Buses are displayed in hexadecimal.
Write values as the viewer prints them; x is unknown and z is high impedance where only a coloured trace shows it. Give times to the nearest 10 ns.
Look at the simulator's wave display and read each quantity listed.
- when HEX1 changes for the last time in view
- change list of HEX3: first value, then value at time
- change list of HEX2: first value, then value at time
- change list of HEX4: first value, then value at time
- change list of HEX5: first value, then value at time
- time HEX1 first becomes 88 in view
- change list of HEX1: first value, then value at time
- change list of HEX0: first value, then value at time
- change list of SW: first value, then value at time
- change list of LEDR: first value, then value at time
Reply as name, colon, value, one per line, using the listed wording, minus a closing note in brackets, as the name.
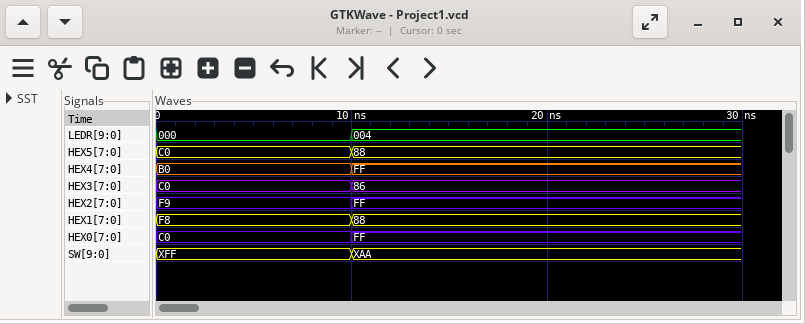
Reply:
when HEX1 changes for the last time in view: 10 ns
change list of HEX3: first value, then value at time: C0, 86 at 10 ns
change list of HEX2: first value, then value at time: F9, FF at 10 ns
change list of HEX4: first value, then value at time: B0, FF at 10 ns
change list of HEX5: first value, then value at time: C0, 88 at 10 ns
time HEX1 first becomes 88 in view: 10 ns
change list of HEX1: first value, then value at time: F8, 88 at 10 ns
change list of HEX0: first value, then value at time: C0, FF at 10 ns
change list of SW: first value, then value at time: XFF, XAA at 10 ns
change list of LEDR: first value, then value at time: 000, 004 at 10 ns
